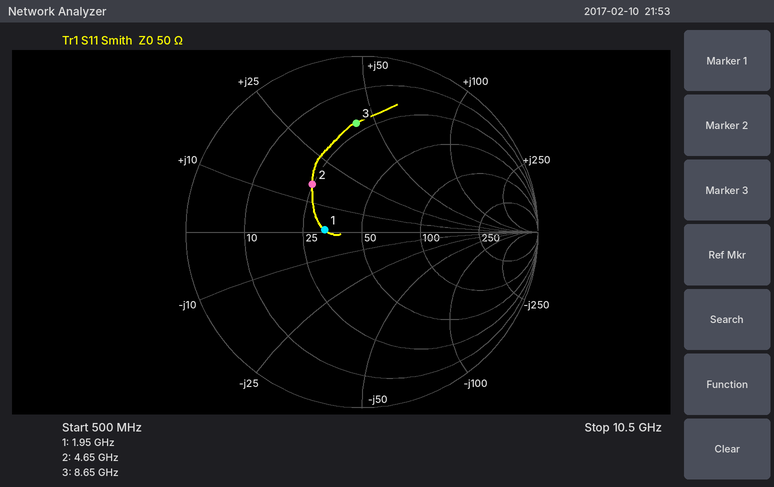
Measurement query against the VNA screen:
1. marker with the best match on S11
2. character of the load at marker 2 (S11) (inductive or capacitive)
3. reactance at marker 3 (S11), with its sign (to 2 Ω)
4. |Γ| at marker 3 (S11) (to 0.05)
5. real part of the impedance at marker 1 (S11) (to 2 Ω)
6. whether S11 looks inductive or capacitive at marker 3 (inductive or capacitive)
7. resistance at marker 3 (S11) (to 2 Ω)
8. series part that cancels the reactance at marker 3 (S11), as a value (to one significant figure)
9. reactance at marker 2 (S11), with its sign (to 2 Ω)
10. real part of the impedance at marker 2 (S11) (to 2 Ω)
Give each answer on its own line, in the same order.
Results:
marker 1
inductive
+42 Ω
0.60
32 Ω
inductive
22 Ω
400 fF
+16 Ω
24 Ω
